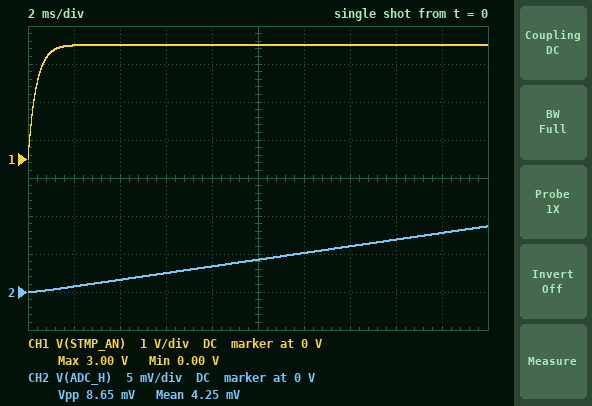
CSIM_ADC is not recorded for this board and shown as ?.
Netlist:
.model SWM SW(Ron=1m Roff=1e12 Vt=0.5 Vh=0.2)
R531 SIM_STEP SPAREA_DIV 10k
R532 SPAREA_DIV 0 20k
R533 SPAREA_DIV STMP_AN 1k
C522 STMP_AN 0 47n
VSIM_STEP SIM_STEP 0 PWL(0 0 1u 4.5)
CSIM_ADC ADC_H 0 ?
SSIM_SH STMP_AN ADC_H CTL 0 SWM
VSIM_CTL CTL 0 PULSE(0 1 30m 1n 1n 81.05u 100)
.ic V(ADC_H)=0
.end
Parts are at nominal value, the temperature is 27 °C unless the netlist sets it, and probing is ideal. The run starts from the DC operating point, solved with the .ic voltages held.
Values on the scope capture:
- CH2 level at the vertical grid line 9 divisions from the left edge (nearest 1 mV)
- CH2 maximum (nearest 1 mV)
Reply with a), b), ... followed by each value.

a) 8 mV
b) 9 mV
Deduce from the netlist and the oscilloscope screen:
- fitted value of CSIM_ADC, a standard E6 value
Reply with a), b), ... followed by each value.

a) 6.8 pF
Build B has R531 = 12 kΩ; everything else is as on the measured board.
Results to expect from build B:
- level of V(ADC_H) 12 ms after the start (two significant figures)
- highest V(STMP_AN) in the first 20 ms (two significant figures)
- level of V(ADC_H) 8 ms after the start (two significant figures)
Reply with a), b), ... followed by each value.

a) 4.8 mV
b) 2.8 V
c) 3.1 mV
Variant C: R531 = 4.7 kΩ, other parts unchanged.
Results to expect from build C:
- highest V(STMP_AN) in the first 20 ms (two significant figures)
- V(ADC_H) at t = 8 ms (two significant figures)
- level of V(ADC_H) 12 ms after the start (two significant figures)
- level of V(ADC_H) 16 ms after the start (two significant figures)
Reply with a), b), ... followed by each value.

a) 3.6 V
b) 4.2 mV
c) 6.3 mV
d) 8.4 mV
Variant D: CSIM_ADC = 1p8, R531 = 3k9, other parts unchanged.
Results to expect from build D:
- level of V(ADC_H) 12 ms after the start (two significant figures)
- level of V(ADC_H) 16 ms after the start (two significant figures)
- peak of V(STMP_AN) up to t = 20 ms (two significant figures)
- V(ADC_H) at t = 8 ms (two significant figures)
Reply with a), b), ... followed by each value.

a) 25 mV
b) 33 mV
c) 3.8 V
d) 16 mV
